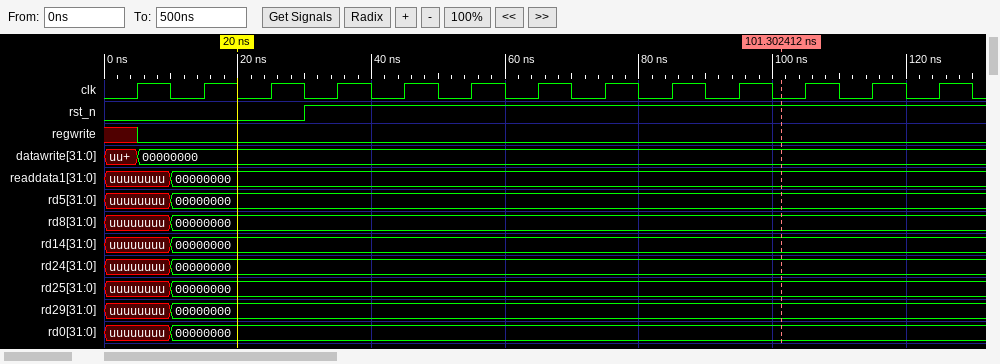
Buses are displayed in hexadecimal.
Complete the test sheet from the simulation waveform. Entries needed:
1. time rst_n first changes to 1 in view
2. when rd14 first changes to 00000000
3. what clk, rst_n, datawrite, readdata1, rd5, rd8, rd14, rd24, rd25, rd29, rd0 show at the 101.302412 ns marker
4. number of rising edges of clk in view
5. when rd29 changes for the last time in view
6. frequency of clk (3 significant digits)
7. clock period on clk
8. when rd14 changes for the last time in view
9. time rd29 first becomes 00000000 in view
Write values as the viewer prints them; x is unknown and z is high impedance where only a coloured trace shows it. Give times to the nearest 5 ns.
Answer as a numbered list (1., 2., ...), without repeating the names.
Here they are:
1. 30 ns
2. 10 ns
3. clk=0, rst_n=1, datawrite=00000000, readdata1=00000000, rd5=00000000, rd8=00000000, rd14=00000000, rd24=00000000, rd25=00000000, rd29=00000000, rd0=00000000
4. 13
5. 10 ns
6. 100 MHz
7. 10 ns
8. 10 ns
9. 10 ns
